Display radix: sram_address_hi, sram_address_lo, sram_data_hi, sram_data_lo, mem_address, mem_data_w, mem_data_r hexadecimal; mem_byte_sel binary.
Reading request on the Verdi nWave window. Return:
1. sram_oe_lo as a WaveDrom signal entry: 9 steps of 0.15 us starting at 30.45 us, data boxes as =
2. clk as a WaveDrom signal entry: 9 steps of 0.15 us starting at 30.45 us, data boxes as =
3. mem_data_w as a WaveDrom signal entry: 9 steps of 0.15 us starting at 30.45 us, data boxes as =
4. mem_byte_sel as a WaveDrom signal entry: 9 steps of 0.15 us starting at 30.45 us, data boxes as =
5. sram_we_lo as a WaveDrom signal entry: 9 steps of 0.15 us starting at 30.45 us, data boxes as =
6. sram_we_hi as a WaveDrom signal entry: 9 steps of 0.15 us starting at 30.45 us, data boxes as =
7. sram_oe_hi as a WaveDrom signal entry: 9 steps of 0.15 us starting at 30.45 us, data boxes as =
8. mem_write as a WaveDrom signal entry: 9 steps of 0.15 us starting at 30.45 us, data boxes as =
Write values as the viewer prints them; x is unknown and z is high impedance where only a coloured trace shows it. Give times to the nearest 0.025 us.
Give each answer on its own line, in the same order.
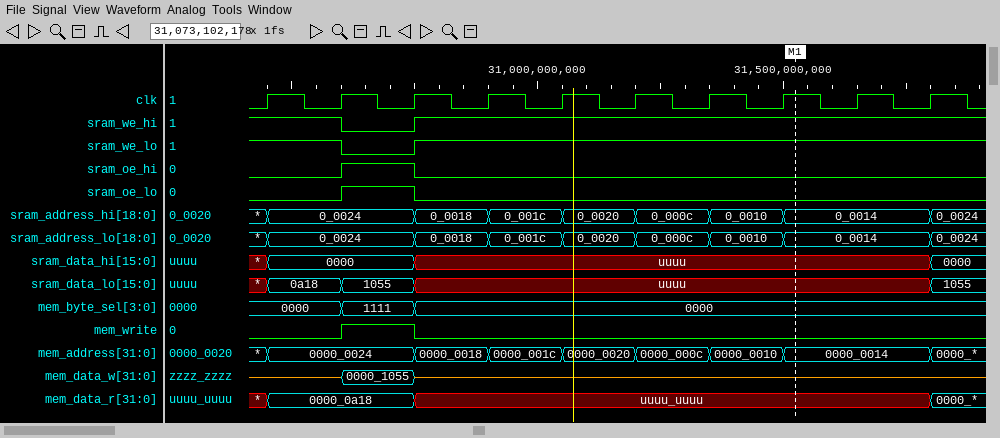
{name: 'sram_oe_lo', wave: '010......'}
{name: 'clk', wave: 'p........'}
{name: 'mem_data_w', wave: 'z=z......', data: '0000_1055'}
{name: 'mem_byte_sel', wave: '===......', data: '0000 1111 0000'}
{name: 'sram_we_lo', wave: '101......'}
{name: 'sram_we_hi', wave: '101......'}
{name: 'sram_oe_hi', wave: '010......'}
{name: 'mem_write', wave: '010......'}
